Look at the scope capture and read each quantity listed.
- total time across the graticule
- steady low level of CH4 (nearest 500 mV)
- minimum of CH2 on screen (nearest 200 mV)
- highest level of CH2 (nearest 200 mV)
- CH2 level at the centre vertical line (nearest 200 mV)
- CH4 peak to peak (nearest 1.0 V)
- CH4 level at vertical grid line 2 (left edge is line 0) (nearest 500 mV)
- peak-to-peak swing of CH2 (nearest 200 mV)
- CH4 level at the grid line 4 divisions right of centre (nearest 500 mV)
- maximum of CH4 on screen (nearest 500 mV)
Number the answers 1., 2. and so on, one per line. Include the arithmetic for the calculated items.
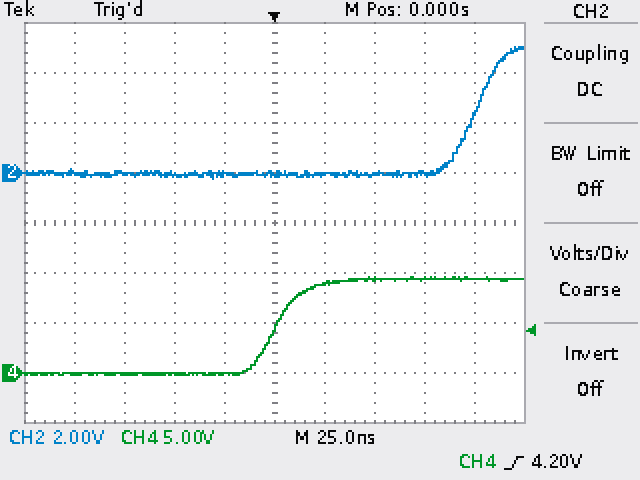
1. 250 ns
2. 0.0 V
3. -200 mV
4. 5.0 V
5. 0.0 V
6. 10.0 V
7. 0.0 V
8. 5.0 V − (-200 mV) = 5.2 V
9. 9.5 V
10. 9.5 V
